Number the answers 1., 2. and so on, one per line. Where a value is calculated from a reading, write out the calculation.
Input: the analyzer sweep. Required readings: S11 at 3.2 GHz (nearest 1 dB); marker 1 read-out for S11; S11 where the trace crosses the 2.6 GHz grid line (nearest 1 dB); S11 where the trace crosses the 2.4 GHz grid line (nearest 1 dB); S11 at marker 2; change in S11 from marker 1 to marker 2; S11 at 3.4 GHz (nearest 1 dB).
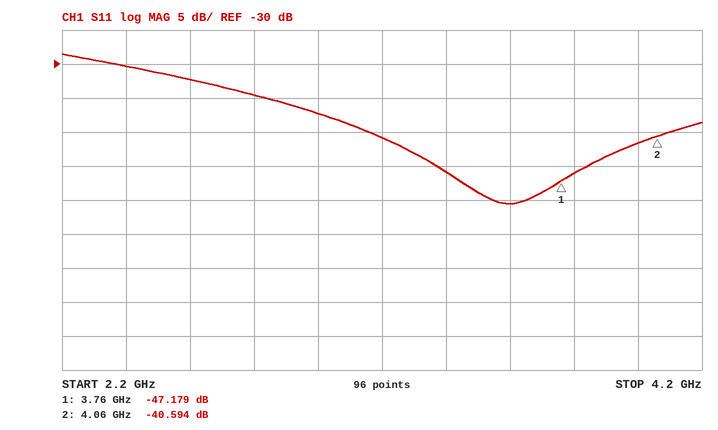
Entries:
1. -41 dB
2. -47.179 dB
3. -32 dB
4. -30 dB
5. -40.594 dB
6. -40.594 − (-47.179) = 6.585 dB
7. -46 dB
